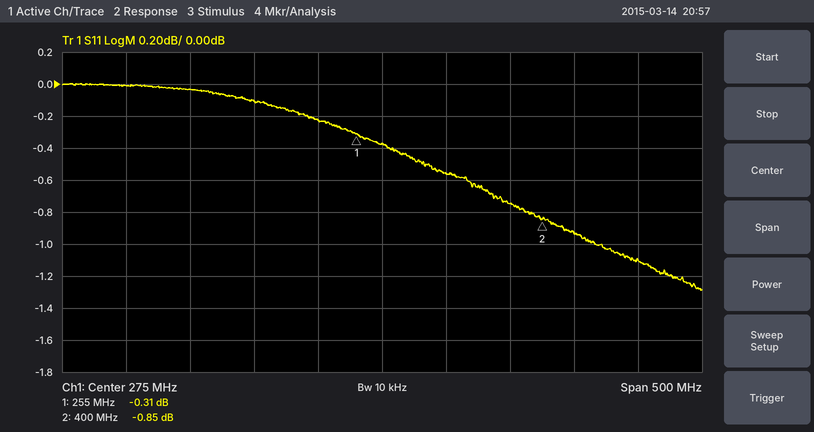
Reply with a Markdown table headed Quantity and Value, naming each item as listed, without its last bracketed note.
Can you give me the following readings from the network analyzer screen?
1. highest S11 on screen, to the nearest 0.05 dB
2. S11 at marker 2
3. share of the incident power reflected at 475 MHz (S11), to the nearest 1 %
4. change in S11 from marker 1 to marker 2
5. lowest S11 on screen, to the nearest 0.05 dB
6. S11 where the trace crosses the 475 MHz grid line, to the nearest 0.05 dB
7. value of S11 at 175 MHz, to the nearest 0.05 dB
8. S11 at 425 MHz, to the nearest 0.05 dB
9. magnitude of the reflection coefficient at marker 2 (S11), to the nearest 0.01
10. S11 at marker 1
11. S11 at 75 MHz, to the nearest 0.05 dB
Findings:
| Quantity | Value |
|---|---|
| highest S11 on screen, to the nearest 0.05 dB | 0.00 dB |
| S11 at marker 2 | -0.85 dB |
| share of the incident power reflected at 475 MHz (S11), to the nearest 1 % | 78 % |
| change in S11 from marker 1 to marker 2 | -0.54 dB |
| lowest S11 on screen, to the nearest 0.05 dB | -1.30 dB |
| S11 where the trace crosses the 475 MHz grid line, to the nearest 0.05 dB | -1.10 dB |
| value of S11 at 175 MHz, to the nearest 0.05 dB | -0.10 dB |
| S11 at 425 MHz, to the nearest 0.05 dB | -0.95 dB |
| magnitude of the reflection coefficient at marker 2 (S11), to the nearest 0.01 | 0.91 |
| S11 at marker 1 | -0.31 dB |
| S11 at 75 MHz, to the nearest 0.05 dB | 0.00 dB |
